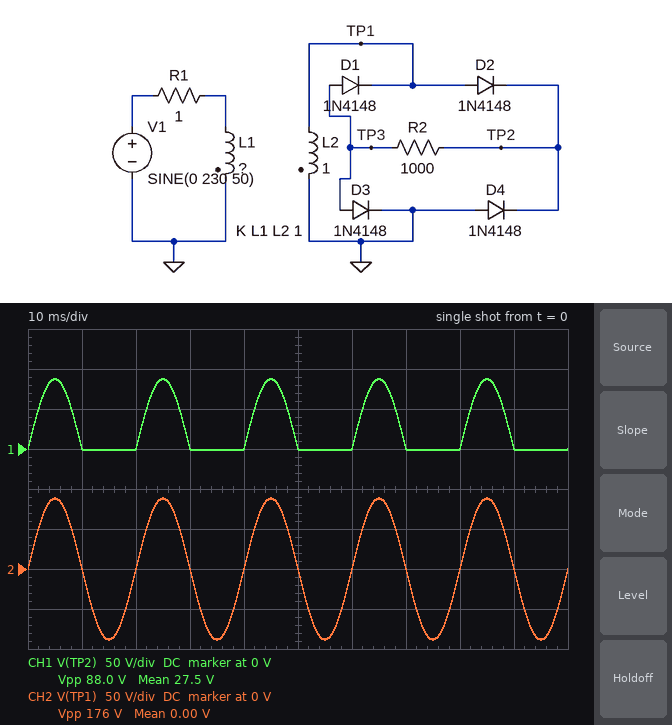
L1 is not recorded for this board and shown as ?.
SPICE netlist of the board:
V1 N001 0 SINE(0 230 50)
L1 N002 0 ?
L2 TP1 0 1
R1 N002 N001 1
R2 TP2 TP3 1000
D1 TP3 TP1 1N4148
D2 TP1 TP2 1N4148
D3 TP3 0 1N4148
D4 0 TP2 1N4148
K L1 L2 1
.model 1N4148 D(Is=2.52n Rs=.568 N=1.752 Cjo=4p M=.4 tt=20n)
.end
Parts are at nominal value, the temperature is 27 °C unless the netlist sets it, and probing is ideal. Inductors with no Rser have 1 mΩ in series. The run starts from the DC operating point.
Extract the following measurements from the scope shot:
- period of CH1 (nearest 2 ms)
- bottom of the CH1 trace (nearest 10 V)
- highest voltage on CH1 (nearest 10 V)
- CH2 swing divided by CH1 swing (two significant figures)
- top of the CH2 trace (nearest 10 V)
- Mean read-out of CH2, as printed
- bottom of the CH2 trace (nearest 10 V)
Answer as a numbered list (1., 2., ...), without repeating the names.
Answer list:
1. 20 ms
2. 0 V
3. 90 V
4. 2.0
5. 90 V
6. 0.00 V
7. -90 V
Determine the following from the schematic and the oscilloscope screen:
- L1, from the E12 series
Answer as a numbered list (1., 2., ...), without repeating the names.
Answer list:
1. 6.8 H
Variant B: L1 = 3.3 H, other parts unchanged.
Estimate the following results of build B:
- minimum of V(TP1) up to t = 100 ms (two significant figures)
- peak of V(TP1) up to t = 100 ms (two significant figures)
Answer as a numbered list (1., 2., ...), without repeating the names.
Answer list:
1. -130 V
2. 130 V
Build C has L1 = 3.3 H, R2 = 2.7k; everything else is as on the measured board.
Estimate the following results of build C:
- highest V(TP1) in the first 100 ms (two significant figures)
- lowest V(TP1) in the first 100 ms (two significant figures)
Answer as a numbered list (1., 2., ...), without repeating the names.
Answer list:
1. 130 V
2. -130 V
